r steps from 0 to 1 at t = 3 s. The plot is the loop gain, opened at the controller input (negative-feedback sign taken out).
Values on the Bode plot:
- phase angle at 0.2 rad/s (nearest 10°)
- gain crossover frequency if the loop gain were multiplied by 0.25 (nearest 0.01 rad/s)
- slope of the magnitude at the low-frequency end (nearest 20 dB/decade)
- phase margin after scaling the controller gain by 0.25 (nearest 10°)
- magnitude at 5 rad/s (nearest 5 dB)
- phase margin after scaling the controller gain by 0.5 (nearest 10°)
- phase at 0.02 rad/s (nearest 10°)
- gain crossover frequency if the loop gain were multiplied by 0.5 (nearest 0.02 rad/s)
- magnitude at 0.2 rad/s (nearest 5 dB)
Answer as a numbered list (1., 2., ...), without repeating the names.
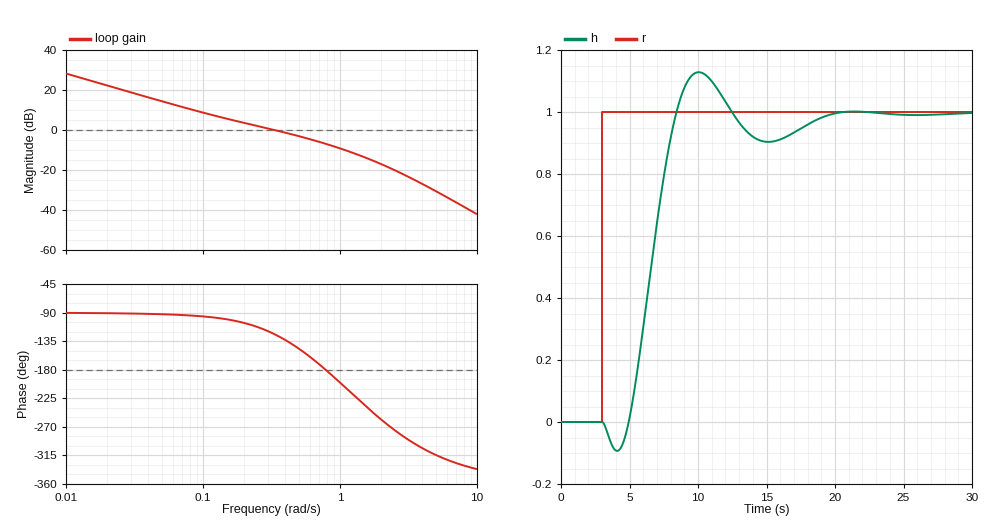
1. -110°
2. 0.07 rad/s
3. -20 dB/decade
4. 90°
5. -30 dB
6. 80°
7. -90°
8. 0.14 rad/s
9. 5 dB
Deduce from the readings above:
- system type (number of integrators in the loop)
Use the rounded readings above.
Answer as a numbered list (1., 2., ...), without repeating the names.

1. 1
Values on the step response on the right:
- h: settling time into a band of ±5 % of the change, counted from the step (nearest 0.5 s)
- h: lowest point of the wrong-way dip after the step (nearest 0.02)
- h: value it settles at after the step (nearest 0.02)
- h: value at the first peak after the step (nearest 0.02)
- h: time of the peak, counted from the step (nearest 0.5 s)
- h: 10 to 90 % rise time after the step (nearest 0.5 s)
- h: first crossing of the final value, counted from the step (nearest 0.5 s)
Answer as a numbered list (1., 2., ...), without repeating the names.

1. 14.5 s
2. -0.10
3. 1.00
4. 1.12
5. 7.0 s
6. 2.5 s
7. 5.5 s
